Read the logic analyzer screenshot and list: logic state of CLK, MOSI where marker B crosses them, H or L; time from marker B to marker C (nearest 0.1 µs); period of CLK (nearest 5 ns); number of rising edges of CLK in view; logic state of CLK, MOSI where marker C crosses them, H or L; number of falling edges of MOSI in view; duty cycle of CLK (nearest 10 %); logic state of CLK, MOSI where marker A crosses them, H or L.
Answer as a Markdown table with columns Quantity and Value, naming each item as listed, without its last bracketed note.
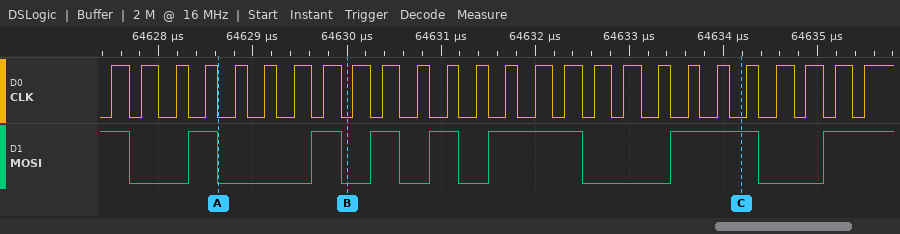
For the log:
| Quantity | Value |
|---|---|
| logic state of CLK, MOSI where marker B crosses them, H or L | CLK=L, MOSI=L |
| time from marker B to marker C | 4.2 µs |
| period of CLK | 320 ns |
| number of rising edges of CLK in view | 26 |
| logic state of CLK, MOSI where marker C crosses them, H or L | CLK=L, MOSI=H |
| number of falling edges of MOSI in view | 7 |
| duty cycle of CLK | 50 % |
| logic state of CLK, MOSI where marker A crosses them, H or L | CLK=L, MOSI=L |
